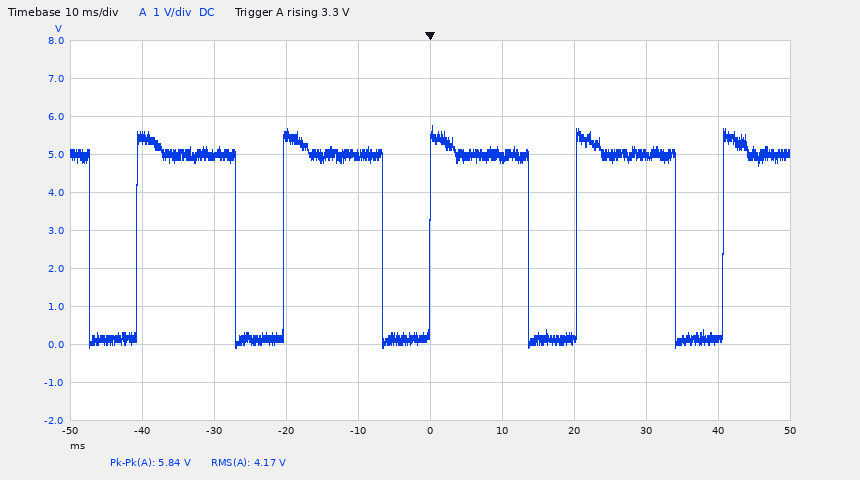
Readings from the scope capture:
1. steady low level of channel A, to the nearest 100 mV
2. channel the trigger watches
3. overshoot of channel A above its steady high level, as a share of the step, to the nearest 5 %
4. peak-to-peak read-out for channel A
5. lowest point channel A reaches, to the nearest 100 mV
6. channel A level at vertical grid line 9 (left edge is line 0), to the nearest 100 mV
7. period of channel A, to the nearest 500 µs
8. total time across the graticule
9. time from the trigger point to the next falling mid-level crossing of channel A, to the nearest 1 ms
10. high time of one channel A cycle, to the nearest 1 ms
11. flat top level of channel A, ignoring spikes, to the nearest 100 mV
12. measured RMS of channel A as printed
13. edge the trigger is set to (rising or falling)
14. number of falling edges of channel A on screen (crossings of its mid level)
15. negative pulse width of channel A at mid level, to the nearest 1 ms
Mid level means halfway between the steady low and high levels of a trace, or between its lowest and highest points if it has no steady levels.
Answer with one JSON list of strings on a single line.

["200 mV", "channel A", "15 %", "5.84 V", "-100 mV", "200 mV", "20.5 ms", "100 ms", "14 ms", "14 ms", "5.0 V", "4.17 V", "rising", "5", "7 ms"]
